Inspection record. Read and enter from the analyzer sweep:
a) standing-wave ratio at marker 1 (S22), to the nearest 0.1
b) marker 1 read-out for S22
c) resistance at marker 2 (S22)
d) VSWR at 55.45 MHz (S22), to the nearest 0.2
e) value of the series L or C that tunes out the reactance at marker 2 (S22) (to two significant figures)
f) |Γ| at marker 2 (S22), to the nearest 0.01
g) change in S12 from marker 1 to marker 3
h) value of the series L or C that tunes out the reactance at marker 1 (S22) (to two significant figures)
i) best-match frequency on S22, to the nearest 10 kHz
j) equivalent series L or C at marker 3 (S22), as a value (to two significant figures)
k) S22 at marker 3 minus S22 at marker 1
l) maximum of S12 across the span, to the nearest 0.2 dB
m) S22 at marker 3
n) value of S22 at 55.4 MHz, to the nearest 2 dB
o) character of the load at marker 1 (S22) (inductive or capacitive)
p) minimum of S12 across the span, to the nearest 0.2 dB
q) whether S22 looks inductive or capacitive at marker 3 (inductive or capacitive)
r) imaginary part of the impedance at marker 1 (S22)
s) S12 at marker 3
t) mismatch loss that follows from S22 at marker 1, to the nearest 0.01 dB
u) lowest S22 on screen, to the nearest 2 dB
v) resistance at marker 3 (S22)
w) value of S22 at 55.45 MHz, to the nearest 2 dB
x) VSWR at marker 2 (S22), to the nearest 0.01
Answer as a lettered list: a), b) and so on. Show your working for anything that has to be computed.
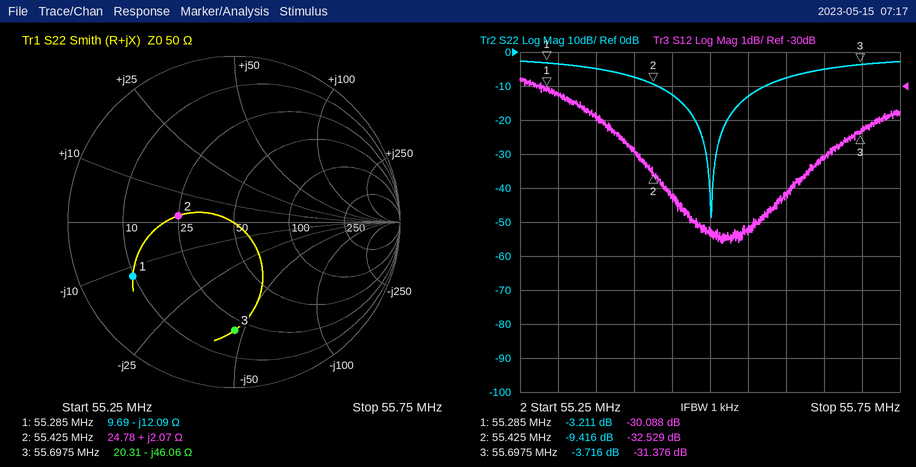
a) 5.5
b) -3.211 dB
c) 24.78 Ω
d) |Γ| = 10^(-12/20) = 0.2512; VSWR = (1 + 0.2512)/(1 − 0.2512) ≈ 1.67, so 1.6 to the nearest 0.2
e) C = 1/(2π × 55.425 MHz × 2.07 Ω) ≈ 1.4 nF
f) 0.34
g) -31.376 − (-30.088) = -1.288 dB
h) L = 12.09 Ω/(2π × 55.285 MHz) ≈ 35 nH
i) 55.50 MHz
j) C = 1/(2π × 55.6975 MHz × 46.06 Ω) ≈ 62 pF
k) -3.716 − (-3.211) = -0.505 dB
l) -29.8 dB
m) -3.716 dB
n) -8 dB
o) capacitive
p) -34.6 dB
q) capacitive
r) -12.09 Ω
s) -31.376 dB
t) −10 log10(1 − 10^(-3.211/10)) ≈ 2.82 dB
u) -48 dB
v) 20.31 Ω
w) -12 dB
x) (1 + 0.3382)/(1 − 0.3382) ≈ 2.02
